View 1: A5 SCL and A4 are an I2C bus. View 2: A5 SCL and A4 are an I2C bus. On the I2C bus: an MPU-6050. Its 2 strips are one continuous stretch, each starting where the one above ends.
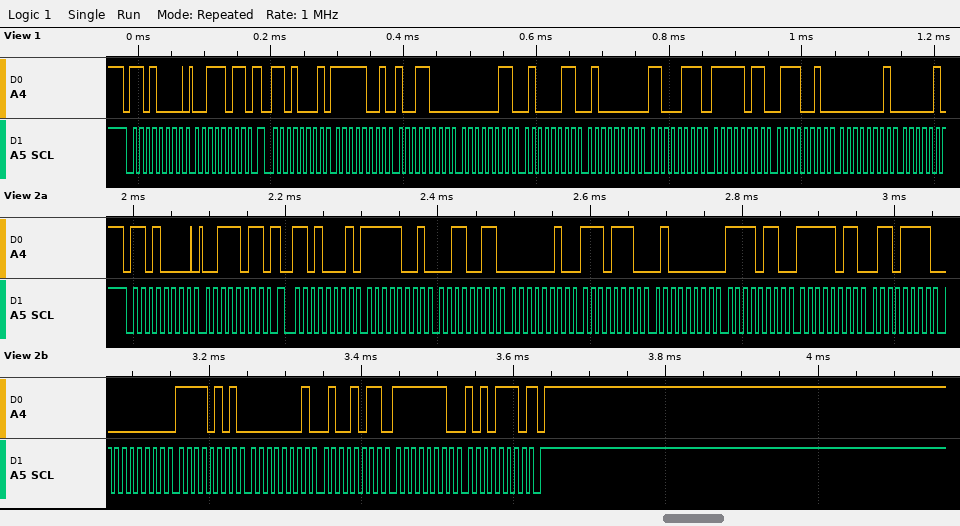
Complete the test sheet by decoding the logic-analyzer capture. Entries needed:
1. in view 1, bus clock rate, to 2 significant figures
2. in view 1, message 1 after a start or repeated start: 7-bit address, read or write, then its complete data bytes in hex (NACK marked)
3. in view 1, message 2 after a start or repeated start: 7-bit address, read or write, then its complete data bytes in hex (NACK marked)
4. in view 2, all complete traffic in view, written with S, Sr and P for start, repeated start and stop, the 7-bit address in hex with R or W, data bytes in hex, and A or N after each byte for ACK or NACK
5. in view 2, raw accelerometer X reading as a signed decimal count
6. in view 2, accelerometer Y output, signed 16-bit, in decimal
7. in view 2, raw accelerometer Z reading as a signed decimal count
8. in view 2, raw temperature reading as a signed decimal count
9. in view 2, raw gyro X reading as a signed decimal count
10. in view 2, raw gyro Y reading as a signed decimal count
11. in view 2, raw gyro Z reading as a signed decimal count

100 kHz
0x68 write: 3B
0x68 read: F9 98 03 43 40 C7 FB 72 01
S 68W A 3B A Sr 68R A F9 A 33 A 02 A EE A 40 A F6 A FB A 6F A 00 A F5 A 01 A 4B A FE A AE N P
-1741
750
16630
-1169
245
331
-338
